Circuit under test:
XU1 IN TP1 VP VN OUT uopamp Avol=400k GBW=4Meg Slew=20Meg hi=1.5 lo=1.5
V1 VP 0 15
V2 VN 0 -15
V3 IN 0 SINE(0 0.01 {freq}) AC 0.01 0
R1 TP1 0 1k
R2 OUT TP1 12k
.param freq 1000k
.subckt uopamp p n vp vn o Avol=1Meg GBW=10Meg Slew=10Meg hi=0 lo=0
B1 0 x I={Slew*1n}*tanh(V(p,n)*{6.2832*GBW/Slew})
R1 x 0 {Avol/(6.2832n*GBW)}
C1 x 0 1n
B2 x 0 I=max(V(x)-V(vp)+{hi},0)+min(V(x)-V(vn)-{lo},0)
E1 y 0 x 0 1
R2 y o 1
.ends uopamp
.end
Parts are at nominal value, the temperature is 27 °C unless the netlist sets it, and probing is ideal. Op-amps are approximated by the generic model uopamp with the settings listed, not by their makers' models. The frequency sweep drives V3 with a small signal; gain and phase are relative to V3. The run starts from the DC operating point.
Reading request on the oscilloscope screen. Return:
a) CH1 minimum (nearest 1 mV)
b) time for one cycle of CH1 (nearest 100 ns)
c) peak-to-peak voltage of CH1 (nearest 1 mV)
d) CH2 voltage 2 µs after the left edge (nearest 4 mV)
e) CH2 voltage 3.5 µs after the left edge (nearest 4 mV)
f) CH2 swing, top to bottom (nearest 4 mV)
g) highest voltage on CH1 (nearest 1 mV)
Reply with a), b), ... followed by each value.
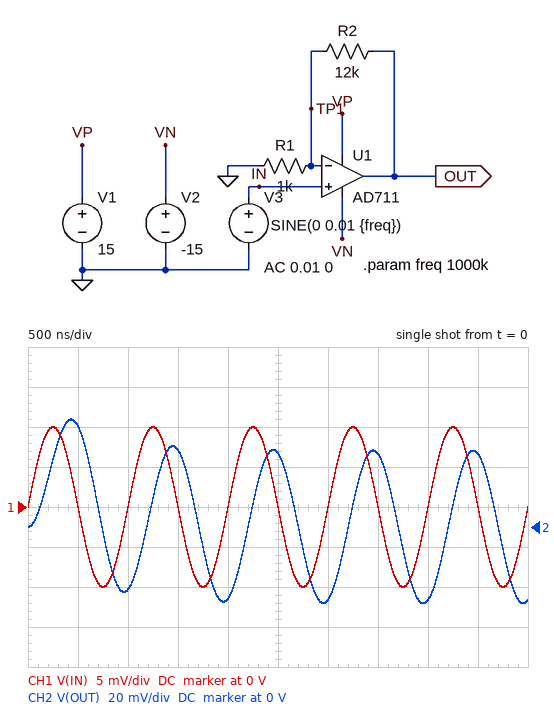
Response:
a) -10 mV
b) 1.0 µs
c) 20 mV
d) -36 mV
e) 36 mV
f) 92 mV
g) 10 mV
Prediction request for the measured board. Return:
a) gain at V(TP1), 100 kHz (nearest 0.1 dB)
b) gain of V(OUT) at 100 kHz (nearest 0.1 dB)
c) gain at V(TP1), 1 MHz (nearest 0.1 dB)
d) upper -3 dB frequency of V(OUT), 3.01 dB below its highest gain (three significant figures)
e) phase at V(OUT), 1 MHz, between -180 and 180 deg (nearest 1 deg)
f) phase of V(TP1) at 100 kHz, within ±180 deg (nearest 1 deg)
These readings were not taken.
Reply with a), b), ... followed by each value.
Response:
a) -0.4 dB
b) 21.8 dB
c) -10.6 dB
d) 308 kHz
e) -73 deg
f) -18 deg
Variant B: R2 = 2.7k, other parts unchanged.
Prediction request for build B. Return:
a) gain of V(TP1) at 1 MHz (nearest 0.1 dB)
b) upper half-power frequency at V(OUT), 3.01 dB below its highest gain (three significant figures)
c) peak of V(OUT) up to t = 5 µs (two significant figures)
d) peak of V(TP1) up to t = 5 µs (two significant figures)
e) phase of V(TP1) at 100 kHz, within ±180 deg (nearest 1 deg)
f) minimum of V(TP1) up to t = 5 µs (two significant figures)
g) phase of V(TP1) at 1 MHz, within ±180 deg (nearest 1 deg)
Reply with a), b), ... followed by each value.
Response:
a) -2.7 dB
b) 1.08 MHz
c) 29 mV
d) 7.8 mV
e) -5 deg
f) -7.3 mV
g) -43 deg
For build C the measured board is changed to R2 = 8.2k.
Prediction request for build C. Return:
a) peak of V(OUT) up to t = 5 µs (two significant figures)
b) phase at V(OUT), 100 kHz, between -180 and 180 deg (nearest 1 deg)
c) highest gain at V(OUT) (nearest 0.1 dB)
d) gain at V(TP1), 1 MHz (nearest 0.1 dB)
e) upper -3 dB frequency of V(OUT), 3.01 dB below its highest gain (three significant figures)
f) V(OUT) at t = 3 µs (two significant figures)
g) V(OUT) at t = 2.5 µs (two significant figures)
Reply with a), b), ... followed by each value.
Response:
a) 47 mV
b) -13 deg
c) 19.3 dB
d) -8.0 dB
e) 435 kHz
f) -34 mV
g) 34 mV
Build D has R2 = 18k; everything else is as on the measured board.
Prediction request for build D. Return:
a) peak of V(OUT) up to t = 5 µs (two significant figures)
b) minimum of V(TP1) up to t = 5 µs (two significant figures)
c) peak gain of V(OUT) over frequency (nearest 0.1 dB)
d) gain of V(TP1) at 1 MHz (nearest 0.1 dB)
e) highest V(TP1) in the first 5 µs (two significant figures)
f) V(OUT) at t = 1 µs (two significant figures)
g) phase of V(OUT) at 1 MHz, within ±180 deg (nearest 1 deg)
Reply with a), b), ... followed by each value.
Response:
a) 60 mV
b) -2.1 mV
c) 25.6 dB
d) -13.7 dB
e) 3.2 mV
f) -28 mV
g) -78 deg
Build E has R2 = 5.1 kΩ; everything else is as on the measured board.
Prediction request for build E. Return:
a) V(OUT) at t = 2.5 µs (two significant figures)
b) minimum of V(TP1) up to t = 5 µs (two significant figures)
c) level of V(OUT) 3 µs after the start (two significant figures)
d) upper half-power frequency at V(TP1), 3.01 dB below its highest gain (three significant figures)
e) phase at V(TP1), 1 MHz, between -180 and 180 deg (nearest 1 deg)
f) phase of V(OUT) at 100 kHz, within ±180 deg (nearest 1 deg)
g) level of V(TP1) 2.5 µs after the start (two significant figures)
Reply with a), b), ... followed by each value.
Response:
a) 28 mV
b) -5.5 mV
c) -28 mV
d) 656 kHz
e) -57 deg
f) -9 deg
g) 4.6 mV
